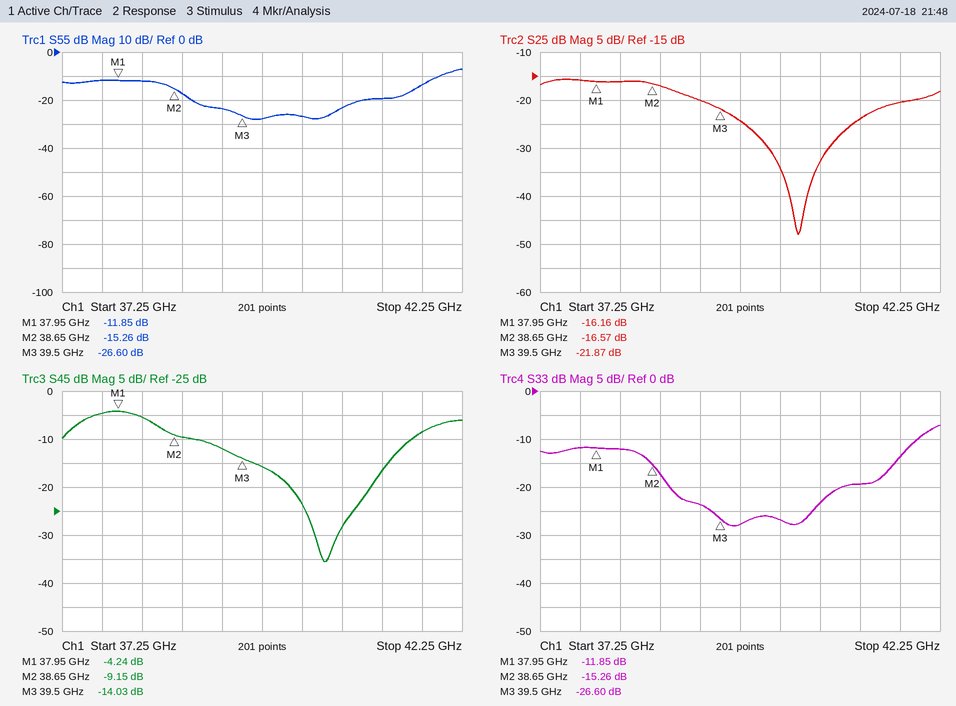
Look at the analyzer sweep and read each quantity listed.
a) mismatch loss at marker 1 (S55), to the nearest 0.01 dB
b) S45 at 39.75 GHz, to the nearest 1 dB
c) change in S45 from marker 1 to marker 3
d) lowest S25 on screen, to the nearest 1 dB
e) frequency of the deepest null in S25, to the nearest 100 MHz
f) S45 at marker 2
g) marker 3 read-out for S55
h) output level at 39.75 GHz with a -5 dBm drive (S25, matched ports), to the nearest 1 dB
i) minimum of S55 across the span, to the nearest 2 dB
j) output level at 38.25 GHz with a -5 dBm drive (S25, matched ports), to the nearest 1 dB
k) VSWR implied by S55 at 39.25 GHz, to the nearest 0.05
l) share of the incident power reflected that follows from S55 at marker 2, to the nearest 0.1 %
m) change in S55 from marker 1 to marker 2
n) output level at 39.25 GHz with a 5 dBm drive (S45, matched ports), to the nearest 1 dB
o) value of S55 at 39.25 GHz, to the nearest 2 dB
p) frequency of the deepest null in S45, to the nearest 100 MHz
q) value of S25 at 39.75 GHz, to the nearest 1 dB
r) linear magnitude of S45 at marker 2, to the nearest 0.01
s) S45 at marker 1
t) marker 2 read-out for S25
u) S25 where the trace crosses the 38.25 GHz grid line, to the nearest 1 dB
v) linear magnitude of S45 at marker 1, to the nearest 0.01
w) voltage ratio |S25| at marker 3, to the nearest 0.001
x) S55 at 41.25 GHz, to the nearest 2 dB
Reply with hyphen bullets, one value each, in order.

- 0.29 dB
- -16 dB
- -9.79 dB
- -48 dB
- 40.5 GHz
- -9.15 dB
- -26.60 dB
- -29 dBm
- -28 dB
- -21 dBm
- 1.15
- 3.0 %
- -3.41 dB
- -7 dBm
- -24 dB
- 40.5 GHz
- -24 dB
- 0.35
- -4.24 dB
- -16.57 dB
- -16 dB
- 0.61
- 0.081
- -20 dB
